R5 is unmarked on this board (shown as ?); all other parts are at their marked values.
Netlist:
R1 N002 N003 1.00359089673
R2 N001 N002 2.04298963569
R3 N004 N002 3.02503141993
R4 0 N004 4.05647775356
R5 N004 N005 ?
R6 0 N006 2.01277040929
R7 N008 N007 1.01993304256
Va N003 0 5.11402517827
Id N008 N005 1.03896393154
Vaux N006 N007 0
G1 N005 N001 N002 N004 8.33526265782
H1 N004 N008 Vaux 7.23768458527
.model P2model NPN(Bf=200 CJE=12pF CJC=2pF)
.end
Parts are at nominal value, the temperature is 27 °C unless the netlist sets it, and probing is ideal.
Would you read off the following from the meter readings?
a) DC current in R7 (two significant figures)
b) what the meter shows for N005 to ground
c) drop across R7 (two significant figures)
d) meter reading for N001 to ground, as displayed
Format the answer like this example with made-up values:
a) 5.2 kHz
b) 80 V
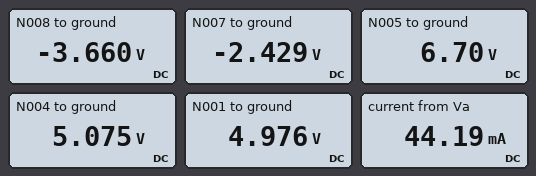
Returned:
a) 1.2 A
b) 6.70 V
c) 1.2 V
d) 4.976 V
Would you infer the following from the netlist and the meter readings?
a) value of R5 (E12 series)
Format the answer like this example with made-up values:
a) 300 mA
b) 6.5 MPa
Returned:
a) 1.5 Ω
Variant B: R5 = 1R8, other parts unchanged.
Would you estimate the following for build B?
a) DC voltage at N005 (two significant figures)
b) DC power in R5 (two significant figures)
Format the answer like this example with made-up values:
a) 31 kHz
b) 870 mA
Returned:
a) 7.0 V
b) 2.1 W
